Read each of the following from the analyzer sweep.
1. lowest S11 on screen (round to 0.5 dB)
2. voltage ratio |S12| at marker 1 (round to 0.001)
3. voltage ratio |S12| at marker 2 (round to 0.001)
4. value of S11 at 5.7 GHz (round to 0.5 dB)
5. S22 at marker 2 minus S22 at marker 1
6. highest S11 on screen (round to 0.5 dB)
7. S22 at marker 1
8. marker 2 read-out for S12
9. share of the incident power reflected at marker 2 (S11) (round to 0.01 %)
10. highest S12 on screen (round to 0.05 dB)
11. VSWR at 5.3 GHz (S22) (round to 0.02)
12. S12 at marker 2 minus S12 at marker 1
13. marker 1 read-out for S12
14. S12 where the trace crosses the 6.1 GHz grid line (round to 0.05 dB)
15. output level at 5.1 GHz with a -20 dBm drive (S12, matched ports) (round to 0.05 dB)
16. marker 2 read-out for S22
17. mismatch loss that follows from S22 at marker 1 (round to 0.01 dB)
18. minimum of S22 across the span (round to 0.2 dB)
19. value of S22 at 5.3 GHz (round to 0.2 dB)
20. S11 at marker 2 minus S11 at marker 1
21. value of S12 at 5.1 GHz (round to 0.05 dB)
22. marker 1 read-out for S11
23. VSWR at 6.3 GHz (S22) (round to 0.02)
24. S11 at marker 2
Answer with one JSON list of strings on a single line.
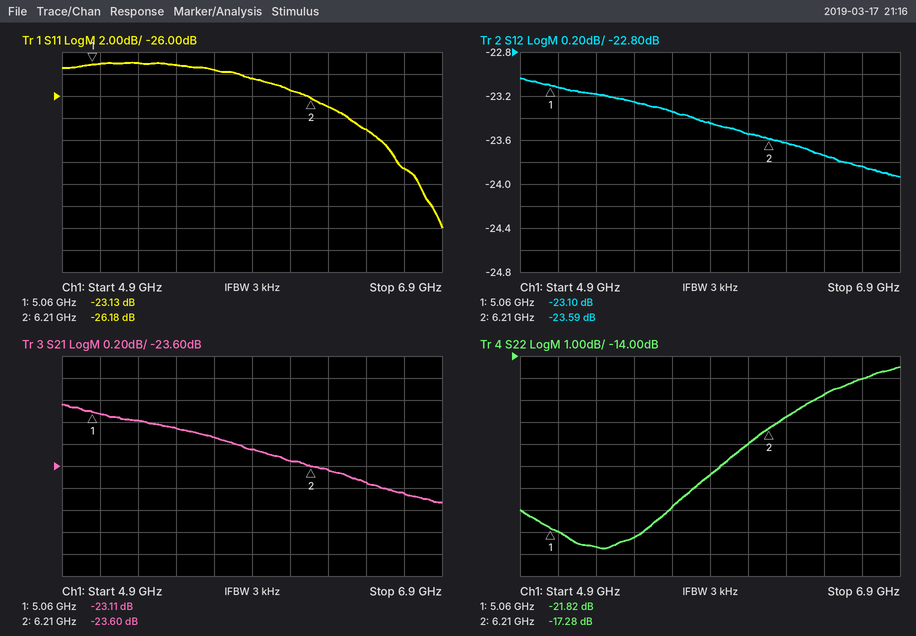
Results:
["-38.0 dB", "0.070", "0.066", "-23.5 dB", "4.54 dB", "-23.0 dB", "-21.82 dB", "-23.59 dB", "0.24 %", "-23.05 dB", "1.16", "-0.49 dB", "-23.10 dB", "-23.55 dB", "-43.10 dBm", "-17.28 dB", "0.03 dB", "-22.8 dB", "-22.6 dB", "-3.05 dB", "-23.10 dB", "-23.13 dB", "1.34", "-26.18 dB"]
